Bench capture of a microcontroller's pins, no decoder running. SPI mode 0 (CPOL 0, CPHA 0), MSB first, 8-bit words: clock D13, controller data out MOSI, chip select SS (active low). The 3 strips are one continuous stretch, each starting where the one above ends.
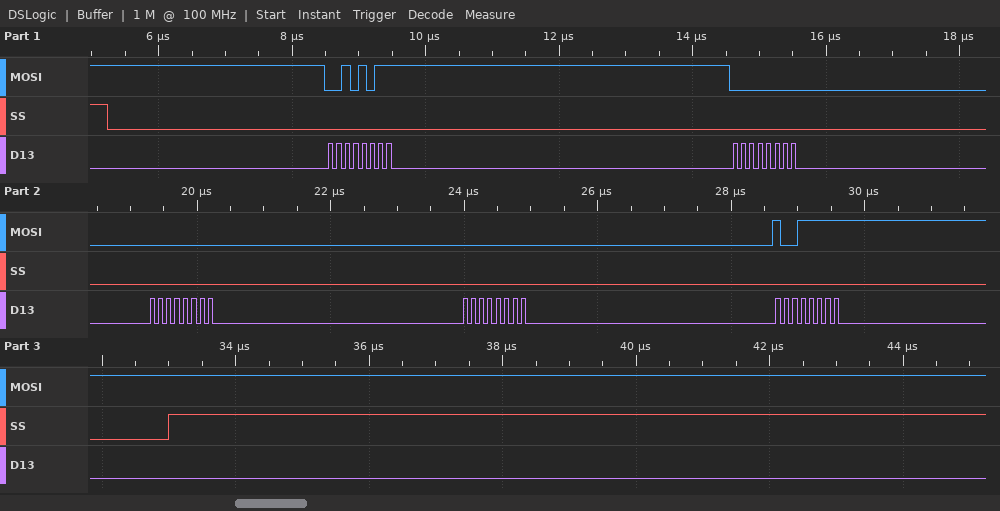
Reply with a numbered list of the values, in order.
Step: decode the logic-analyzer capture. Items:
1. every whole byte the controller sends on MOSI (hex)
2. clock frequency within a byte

1. 0x2B 0x00 0x00 0x00 0x9F
2. 8 MHz
